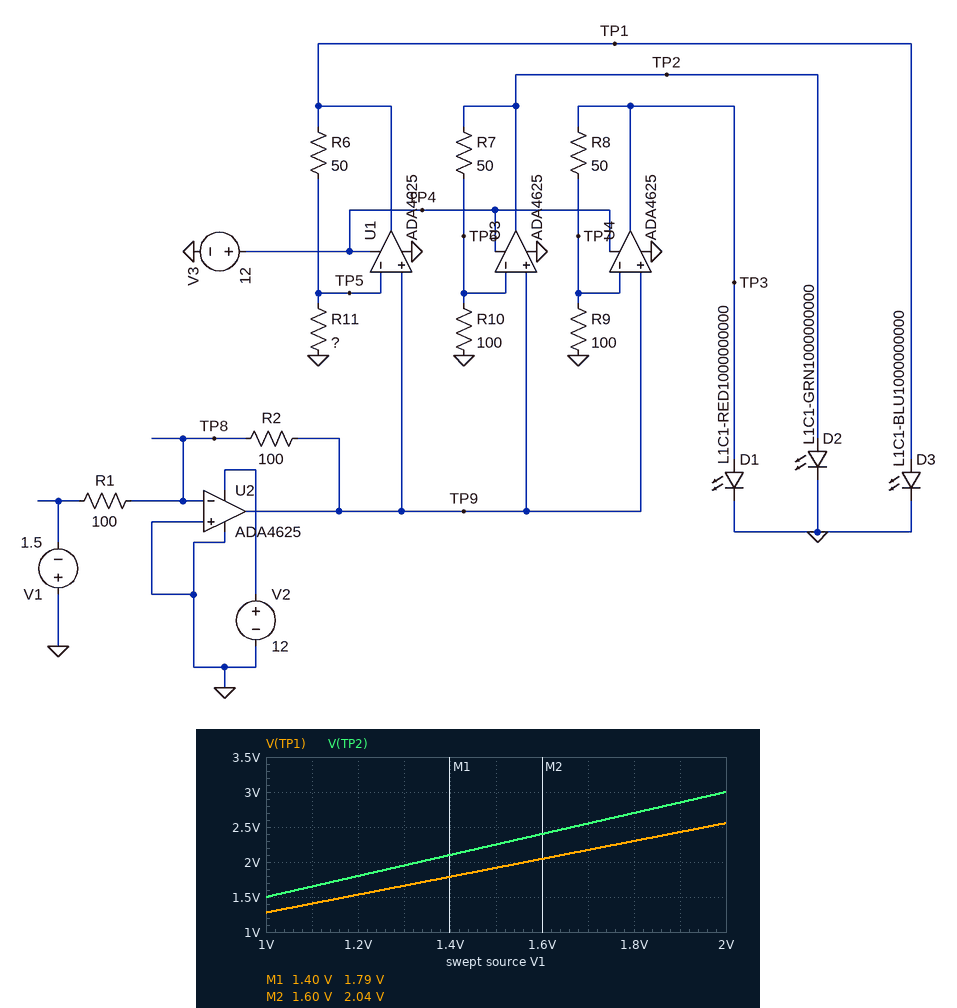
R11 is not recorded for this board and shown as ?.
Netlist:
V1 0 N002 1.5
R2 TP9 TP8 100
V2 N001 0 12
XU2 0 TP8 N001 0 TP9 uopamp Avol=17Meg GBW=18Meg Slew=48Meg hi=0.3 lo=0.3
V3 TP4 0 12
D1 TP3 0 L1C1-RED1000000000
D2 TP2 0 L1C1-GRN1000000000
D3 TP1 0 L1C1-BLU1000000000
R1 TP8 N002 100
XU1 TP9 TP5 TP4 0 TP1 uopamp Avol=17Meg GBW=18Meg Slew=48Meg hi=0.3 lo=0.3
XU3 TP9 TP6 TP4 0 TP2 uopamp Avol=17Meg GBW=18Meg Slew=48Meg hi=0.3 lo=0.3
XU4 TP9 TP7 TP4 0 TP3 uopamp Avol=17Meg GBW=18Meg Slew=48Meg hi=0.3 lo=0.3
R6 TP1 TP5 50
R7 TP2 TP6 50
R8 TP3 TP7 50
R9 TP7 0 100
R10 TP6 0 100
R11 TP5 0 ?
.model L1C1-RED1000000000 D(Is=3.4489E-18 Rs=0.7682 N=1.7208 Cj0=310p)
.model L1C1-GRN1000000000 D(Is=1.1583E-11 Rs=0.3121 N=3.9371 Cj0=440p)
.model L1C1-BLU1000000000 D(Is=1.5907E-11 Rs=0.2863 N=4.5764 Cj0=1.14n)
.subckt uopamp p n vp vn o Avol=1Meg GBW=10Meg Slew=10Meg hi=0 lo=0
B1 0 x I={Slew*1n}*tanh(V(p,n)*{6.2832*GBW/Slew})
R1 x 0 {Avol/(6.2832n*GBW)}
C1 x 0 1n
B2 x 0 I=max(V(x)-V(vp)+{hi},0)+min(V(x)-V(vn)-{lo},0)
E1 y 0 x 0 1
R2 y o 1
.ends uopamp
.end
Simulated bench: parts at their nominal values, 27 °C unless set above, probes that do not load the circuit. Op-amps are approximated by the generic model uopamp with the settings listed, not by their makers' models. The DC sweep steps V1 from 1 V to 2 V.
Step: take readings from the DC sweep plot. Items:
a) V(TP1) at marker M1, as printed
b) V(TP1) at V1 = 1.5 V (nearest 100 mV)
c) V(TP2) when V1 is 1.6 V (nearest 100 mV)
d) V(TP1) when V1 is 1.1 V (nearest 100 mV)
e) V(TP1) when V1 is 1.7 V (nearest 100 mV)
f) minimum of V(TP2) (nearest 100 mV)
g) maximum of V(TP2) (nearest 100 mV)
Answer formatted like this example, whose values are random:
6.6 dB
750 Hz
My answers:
1.79 V
1.9 V
2.4 V
1.4 V
2.2 V
1.5 V
3.0 V
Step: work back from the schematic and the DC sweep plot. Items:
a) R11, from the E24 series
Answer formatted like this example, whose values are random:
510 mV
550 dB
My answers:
180 Ω
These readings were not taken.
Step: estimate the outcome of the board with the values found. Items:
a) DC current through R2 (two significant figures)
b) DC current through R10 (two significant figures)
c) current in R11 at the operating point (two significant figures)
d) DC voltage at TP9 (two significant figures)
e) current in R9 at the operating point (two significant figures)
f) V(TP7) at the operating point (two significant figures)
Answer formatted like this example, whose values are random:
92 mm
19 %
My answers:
15 mA
15 mA
8.3 mA
1.5 V
15 mA
1.5 V
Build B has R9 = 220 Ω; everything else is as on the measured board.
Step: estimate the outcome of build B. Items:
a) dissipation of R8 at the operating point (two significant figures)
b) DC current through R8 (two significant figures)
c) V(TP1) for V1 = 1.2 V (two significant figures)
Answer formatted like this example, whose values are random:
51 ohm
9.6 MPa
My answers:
2.3 mW
6.8 mA
1.5 V
